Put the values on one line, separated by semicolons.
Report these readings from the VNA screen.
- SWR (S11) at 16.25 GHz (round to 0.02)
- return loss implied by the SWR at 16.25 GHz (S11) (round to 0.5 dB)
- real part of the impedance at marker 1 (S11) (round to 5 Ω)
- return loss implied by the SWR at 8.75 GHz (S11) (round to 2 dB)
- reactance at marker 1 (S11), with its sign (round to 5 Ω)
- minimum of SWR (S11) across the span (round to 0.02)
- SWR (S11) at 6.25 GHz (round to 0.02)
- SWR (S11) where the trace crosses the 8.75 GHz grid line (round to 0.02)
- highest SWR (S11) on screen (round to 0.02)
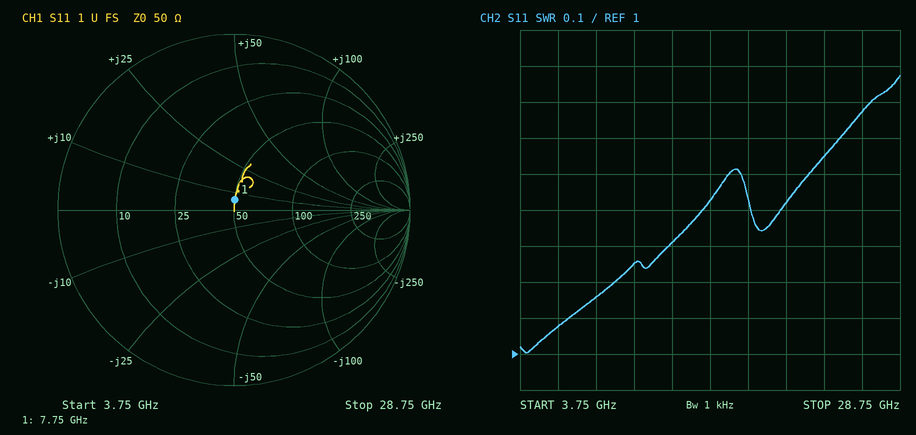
1.42; 15.0 dB; 50 Ω; 22 dB; +5 Ω; 1.00; 1.08; 1.16; 1.78
